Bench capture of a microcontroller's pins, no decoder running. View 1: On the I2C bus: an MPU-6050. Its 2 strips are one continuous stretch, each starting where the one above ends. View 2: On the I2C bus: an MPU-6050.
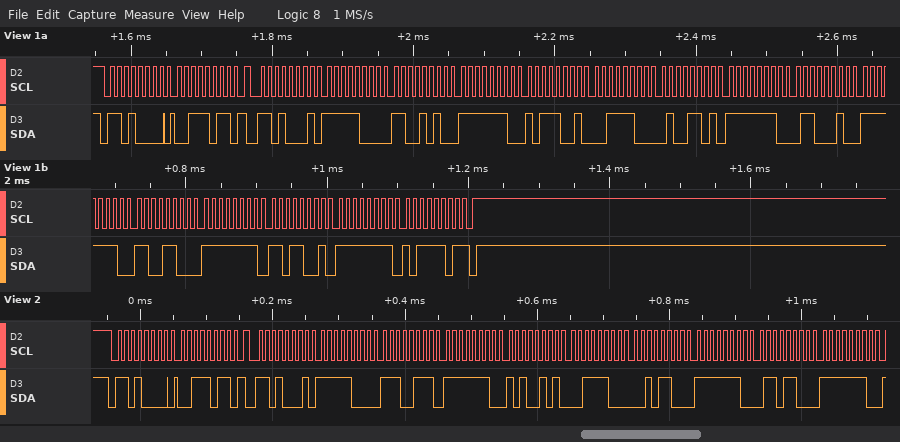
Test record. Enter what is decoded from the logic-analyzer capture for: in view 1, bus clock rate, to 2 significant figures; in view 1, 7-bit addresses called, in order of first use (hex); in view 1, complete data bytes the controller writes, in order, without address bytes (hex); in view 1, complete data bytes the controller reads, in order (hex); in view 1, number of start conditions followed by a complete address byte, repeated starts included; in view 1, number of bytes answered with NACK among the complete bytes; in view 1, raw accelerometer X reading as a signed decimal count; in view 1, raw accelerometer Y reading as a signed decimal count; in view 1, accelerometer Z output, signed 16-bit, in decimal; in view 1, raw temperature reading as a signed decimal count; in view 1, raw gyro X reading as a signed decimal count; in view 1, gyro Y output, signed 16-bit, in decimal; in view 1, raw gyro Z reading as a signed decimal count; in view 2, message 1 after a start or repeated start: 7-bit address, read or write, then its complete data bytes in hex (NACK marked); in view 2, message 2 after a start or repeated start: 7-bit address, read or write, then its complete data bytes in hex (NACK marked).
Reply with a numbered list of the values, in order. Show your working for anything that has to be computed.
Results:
1. 100 kHz
2. 0x68
3. 3B
4. F8 CA FE B9 3C 4D FE 62 FE CC FF D9 FF BD
5. 2
6. 1
7. 0xF8CA = -1846
8. 0xFEB9 = -327
9. 0x3C4D = 15437
10. 0xFE62 = -414
11. 0xFECC = -308
12. 0xFFD9 = -39
13. 0xFFBD = -67
14. 0x68 write: 3B
15. 0x68 read: F8 E7 FE A5 3C 2C FE 6C FE
